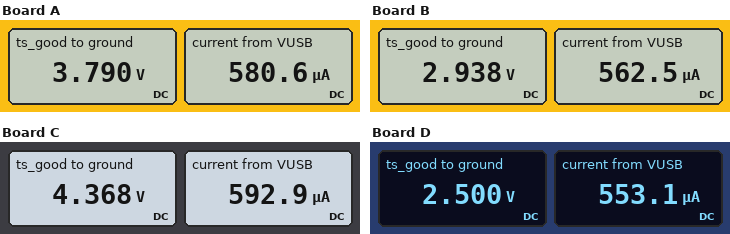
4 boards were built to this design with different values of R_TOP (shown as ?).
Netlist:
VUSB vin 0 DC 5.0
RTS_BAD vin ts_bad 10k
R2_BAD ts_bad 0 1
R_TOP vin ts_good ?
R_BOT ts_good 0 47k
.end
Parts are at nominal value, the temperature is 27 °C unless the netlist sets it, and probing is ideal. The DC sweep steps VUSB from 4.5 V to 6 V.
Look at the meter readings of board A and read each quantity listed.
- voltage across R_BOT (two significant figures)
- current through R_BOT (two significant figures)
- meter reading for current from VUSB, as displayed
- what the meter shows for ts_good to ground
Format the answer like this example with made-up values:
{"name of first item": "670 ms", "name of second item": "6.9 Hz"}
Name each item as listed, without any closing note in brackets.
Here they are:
{"voltage across R_BOT": "3.8 V", "current through R_BOT": "81 µA", "meter reading for current from VUSB, as displayed": "580.6 µA", "what the meter shows for ts_good to ground": "3.790 V"}
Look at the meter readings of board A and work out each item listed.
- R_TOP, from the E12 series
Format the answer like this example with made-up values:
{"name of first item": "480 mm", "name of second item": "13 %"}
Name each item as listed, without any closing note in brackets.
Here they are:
{"R_TOP, from the E12 series": "15 kΩ"}
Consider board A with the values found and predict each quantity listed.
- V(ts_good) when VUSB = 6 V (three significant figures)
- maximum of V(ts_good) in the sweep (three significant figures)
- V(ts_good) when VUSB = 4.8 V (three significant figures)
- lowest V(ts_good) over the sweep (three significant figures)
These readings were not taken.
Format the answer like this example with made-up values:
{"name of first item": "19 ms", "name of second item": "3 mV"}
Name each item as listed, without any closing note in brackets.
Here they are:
{"V(ts_good) when VUSB = 6 V": "4.55 V", "maximum of V(ts_good) in the sweep": "4.55 V", "V(ts_good) when VUSB = 4.8 V": "3.64 V", "lowest V(ts_good) over the sweep": "3.41 V"}
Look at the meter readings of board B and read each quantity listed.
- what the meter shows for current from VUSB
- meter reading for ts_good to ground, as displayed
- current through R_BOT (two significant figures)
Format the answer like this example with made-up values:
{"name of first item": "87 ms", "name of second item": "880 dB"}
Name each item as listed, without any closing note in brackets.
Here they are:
{"what the meter shows for current from VUSB": "562.5 µA", "meter reading for ts_good to ground, as displayed": "2.938 V", "current through R_BOT": "63 µA"}
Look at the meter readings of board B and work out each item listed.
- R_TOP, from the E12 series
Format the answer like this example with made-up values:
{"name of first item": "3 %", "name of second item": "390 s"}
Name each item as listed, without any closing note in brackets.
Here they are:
{"R_TOP, from the E12 series": "33 kΩ"}
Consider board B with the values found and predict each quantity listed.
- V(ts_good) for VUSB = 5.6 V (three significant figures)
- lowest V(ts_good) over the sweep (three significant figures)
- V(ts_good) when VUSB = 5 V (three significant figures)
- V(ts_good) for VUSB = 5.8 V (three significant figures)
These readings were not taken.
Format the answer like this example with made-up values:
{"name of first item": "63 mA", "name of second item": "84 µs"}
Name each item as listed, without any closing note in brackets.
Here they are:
{"V(ts_good) for VUSB = 5.6 V": "3.29 V", "lowest V(ts_good) over the sweep": "2.64 V", "V(ts_good) when VUSB = 5 V": "2.94 V", "V(ts_good) for VUSB = 5.8 V": "3.41 V"}
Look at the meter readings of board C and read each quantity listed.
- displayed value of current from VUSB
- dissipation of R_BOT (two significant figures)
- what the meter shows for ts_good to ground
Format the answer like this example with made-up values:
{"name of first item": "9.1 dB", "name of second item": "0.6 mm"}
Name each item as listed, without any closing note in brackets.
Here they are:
{"displayed value of current from VUSB": "592.9 µA", "dissipation of R_BOT": "410 µW", "what the meter shows for ts_good to ground": "4.368 V"}
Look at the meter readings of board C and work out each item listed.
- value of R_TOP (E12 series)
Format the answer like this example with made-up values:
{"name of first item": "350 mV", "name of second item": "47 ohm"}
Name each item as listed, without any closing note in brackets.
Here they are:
{"value of R_TOP": "6.8 kΩ"}
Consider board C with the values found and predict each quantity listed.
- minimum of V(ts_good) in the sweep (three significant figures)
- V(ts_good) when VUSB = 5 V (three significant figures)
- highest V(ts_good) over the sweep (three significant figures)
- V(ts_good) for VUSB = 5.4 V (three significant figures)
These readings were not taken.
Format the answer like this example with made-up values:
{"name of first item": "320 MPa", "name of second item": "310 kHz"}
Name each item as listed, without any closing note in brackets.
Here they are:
{"minimum of V(ts_good) in the sweep": "3.93 V", "V(ts_good) when VUSB = 5 V": "4.37 V", "highest V(ts_good) over the sweep": "5.24 V", "V(ts_good) for VUSB = 5.4 V": "4.72 V"}
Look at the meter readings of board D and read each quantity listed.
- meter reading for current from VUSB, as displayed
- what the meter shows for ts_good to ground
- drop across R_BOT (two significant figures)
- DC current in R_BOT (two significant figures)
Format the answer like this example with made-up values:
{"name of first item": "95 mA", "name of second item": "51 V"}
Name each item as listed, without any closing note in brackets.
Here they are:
{"meter reading for current from VUSB, as displayed": "553.1 µA", "what the meter shows for ts_good to ground": "2.500 V", "drop across R_BOT": "2.5 V", "DC current in R_BOT": "53 µA"}
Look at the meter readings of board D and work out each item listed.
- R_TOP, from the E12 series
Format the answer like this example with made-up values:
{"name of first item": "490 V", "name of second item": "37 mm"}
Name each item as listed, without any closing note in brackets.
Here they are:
{"R_TOP, from the E12 series": "47 kΩ"}
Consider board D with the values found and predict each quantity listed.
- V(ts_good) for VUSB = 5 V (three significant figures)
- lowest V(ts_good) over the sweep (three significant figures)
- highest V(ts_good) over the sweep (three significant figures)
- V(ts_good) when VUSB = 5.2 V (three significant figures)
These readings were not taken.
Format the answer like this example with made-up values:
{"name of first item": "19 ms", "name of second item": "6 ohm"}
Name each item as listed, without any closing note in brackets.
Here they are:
{"V(ts_good) for VUSB = 5 V": "2.50 V", "lowest V(ts_good) over the sweep": "2.25 V", "highest V(ts_good) over the sweep": "3.00 V", "V(ts_good) when VUSB = 5.2 V": "2.60 V"}
